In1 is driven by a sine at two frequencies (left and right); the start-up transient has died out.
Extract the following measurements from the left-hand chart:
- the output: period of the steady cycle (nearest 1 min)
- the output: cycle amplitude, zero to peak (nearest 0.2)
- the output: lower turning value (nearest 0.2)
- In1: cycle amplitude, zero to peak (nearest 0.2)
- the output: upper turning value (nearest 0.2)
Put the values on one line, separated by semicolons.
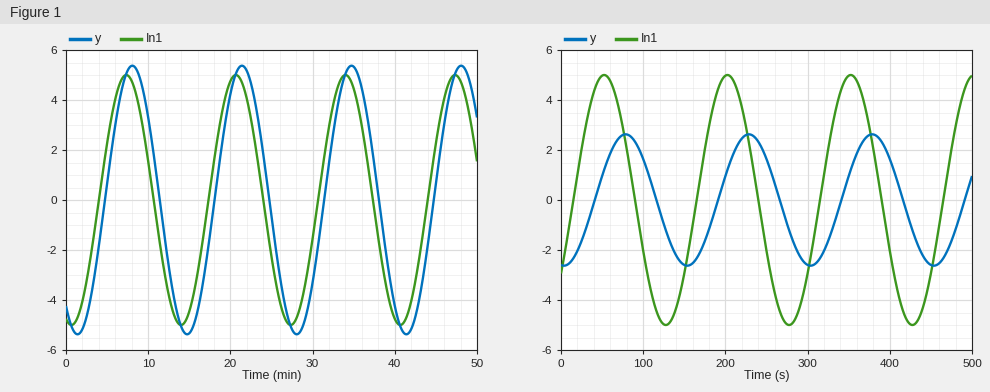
13 min; 5.4; -5.4; 5.0; 5.4
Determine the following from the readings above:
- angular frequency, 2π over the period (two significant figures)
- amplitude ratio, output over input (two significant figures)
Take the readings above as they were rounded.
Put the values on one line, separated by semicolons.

0.48 rad/min; 1.1
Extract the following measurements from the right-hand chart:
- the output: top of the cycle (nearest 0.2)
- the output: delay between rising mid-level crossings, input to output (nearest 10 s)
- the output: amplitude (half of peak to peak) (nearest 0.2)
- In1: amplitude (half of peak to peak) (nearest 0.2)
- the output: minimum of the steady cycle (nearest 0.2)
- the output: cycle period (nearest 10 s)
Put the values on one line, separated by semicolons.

2.6; 30 s; 2.6; 5.0; -2.6; 150 s
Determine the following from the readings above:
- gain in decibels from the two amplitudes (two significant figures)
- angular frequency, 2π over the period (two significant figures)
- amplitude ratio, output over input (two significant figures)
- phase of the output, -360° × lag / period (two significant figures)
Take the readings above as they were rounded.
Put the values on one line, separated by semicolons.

-5.7 dB; 0.042 rad/s; 0.52; -72°
